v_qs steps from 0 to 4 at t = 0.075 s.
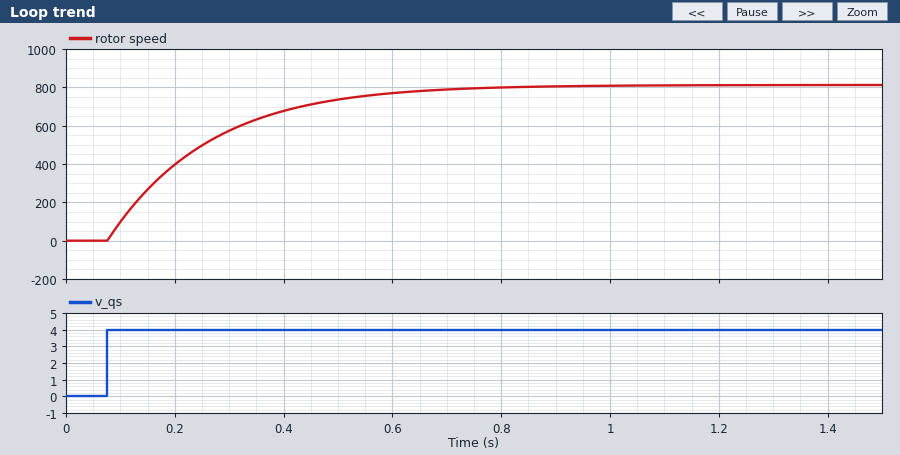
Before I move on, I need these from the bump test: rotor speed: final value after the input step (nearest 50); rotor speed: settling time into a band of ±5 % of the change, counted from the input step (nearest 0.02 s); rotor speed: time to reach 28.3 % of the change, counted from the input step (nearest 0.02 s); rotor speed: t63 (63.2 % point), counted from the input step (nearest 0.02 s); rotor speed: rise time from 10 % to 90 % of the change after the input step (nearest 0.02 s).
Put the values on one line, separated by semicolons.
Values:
800; 0.54 s; 0.06 s; 0.18 s; 0.40 s
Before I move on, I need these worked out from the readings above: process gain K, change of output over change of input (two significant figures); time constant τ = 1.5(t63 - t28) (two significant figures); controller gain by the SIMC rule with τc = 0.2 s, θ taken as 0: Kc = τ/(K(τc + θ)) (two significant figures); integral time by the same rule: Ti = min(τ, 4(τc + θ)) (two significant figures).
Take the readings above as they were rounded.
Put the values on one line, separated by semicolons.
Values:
200; 0.18 s; 0.0045; 0.18 s
